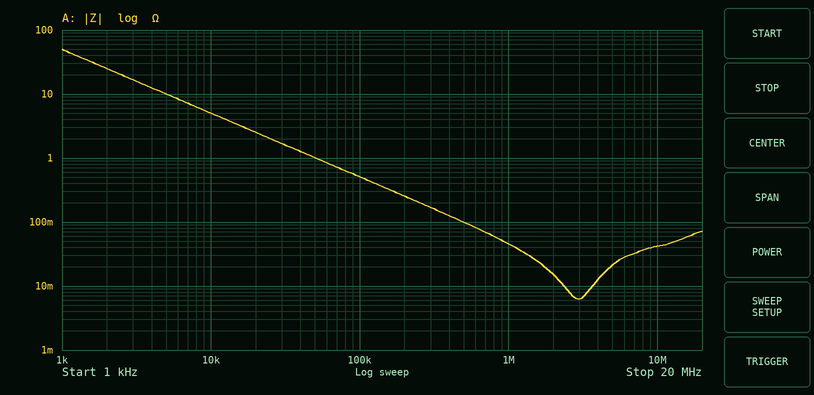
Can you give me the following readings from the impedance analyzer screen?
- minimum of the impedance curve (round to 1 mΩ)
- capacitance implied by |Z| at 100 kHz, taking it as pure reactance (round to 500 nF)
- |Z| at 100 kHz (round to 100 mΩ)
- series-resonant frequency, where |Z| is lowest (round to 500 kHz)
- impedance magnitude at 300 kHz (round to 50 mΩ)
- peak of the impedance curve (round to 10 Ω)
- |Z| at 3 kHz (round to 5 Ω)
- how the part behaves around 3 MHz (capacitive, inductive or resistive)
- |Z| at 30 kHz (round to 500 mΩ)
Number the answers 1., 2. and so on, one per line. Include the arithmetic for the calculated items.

1. 6 mΩ
2. C = 1/(2π × 100 kHz × 500 mΩ) ≈ 3.18 µF, so 3.0 µF to the nearest 500 nF
3. 500 mΩ
4. 3.0 MHz
5. 150 mΩ
6. 50 Ω
7. 15 Ω
8. resistive
9. 1.5 Ω
